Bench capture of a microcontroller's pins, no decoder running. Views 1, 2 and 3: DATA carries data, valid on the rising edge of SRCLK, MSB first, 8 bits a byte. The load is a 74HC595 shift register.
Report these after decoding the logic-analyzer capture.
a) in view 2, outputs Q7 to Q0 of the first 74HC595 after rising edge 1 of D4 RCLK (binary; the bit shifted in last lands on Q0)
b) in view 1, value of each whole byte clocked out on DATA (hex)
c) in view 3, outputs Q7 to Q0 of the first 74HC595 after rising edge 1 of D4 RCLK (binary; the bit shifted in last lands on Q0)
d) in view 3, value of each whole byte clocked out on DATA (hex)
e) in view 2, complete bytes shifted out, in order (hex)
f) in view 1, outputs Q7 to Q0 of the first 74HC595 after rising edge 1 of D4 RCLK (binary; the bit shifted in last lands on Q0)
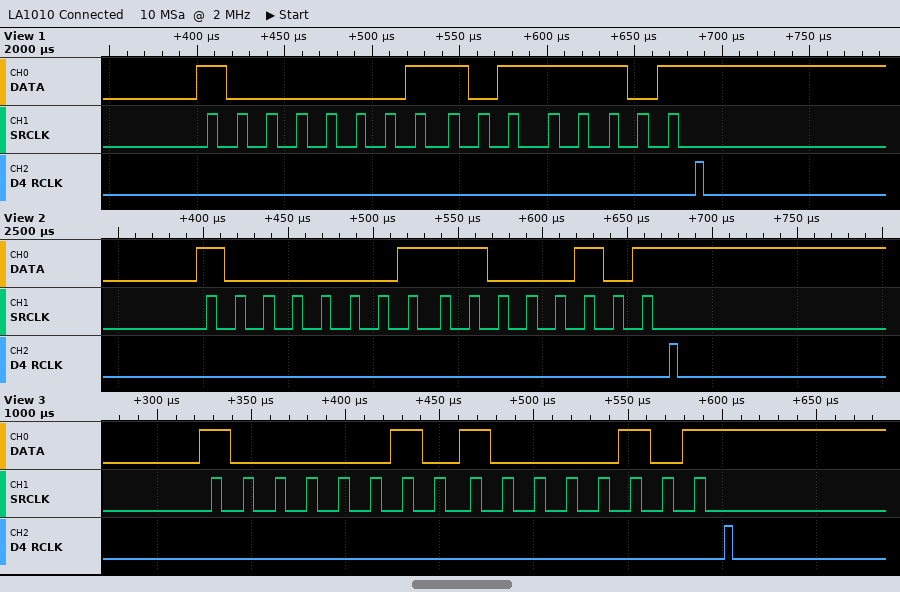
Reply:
11000101
81 BD
10000101
82 85
0x81 0xC5
10111101
